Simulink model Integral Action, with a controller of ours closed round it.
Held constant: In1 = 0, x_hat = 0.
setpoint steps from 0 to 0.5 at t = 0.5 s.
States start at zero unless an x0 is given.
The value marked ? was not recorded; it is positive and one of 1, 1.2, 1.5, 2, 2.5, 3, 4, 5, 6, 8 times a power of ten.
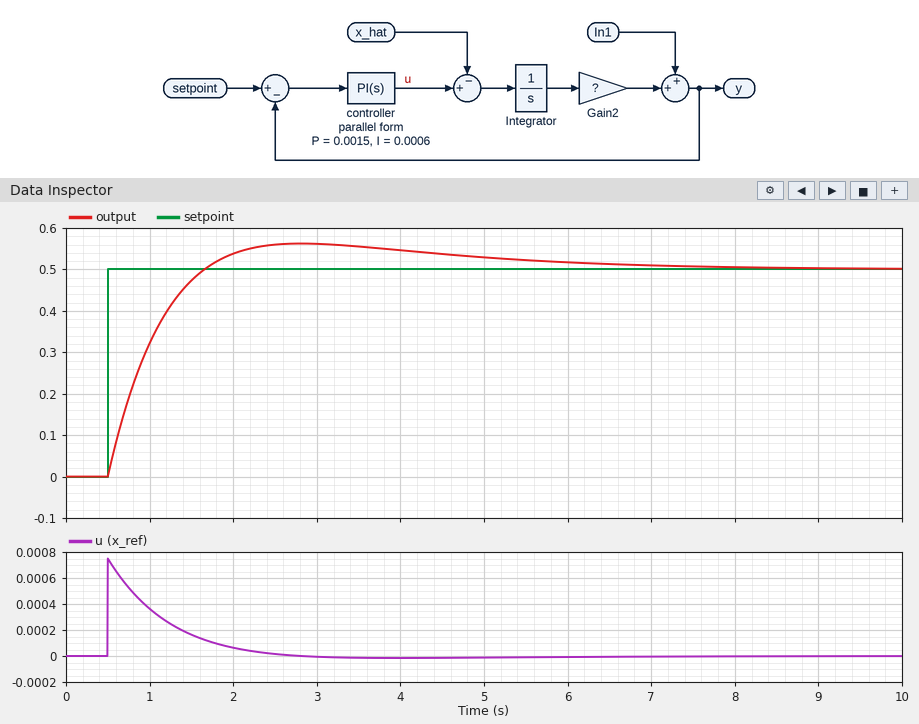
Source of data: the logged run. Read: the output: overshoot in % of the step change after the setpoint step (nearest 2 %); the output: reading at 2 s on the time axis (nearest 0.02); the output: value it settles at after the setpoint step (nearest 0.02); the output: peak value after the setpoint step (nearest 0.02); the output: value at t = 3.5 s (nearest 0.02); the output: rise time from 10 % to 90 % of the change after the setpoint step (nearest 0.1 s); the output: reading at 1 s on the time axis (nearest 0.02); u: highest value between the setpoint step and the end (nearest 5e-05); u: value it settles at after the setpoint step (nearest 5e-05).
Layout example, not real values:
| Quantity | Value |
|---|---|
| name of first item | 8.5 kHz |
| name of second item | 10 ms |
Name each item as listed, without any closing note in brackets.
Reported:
| Quantity | Value |
|---|---|
| the output: overshoot in % of the step change after the setpoint step | 12 % |
| the output: reading at 2 s on the time axis | 0.54 |
| the output: value it settles at after the setpoint step | 0.50 |
| the output: peak value after the setpoint step | 0.56 |
| the output: value at t = 3.5 s | 0.56 |
| the output: rise time from 10 % to 90 % of the change after the setpoint step | 0.8 s |
| the output: reading at 1 s on the time axis | 0.32 |
| u: highest value between the setpoint step and the end | 0.00075 |
| u: value it settles at after the setpoint step | 0.00000 |
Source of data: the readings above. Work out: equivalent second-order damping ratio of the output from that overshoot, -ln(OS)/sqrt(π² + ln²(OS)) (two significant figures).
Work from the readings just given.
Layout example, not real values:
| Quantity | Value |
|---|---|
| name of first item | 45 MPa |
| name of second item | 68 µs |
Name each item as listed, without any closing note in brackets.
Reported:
| Quantity | Value |
|---|---|
| equivalent second-order damping ratio of the output from that overshoot, -ln(OS)/sqrt(π² + ln²(OS)) | 0.56 |
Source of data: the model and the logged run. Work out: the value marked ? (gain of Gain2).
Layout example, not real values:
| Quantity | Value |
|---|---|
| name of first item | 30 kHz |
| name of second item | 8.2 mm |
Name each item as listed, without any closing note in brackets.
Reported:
| Quantity | Value |
|---|---|
| the value marked ? | 1200 |
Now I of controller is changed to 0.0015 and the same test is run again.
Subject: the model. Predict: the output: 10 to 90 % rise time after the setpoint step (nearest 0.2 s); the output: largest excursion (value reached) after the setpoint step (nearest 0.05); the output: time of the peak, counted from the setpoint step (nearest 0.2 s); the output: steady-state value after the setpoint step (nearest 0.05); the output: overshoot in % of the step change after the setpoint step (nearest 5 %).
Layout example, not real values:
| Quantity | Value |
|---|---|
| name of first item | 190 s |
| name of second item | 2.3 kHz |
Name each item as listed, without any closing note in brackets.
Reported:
| Quantity | Value |
|---|---|
| the output: 10 to 90 % rise time after the setpoint step | 0.6 s |
| the output: largest excursion (value reached) after the setpoint step | 0.60 |
| the output: time of the peak, counted from the setpoint step | 1.6 s |
| the output: steady-state value after the setpoint step | 0.50 |
| the output: overshoot in % of the step change after the setpoint step | 20 % |
